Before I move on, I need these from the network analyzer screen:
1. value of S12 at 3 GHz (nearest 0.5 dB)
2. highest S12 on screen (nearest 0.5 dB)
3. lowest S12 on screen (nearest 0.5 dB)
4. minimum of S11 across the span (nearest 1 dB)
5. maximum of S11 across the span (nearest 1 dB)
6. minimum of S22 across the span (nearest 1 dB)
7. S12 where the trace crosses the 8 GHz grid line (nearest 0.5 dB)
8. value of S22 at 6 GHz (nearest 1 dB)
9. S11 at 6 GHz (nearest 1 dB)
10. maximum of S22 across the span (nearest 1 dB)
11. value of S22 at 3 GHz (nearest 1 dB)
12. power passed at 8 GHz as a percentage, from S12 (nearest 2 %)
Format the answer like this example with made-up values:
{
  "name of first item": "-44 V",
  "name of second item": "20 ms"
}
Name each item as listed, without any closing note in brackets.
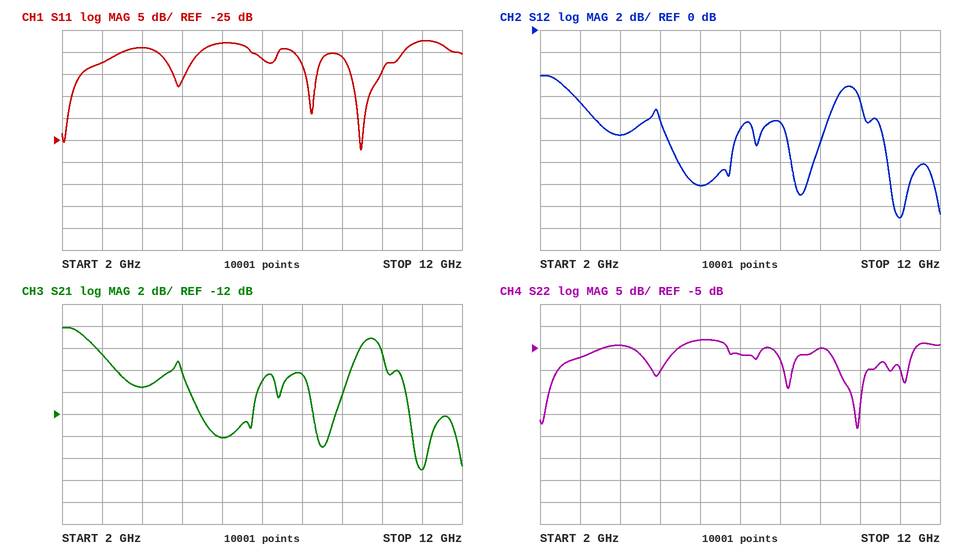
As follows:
{
  "value of S12 at 3 GHz": "-6.5 dB",
  "highest S12 on screen": "-4.0 dB",
  "lowest S12 on screen": "-17.0 dB",
  "minimum of S11 across the span": "-27 dB",
  "maximum of S11 across the span": "-2 dB",
  "minimum of S22 across the span": "-23 dB",
  "S12 where the trace crosses the 8 GHz grid line": "-8.5 dB",
  "value of S22 at 6 GHz": "-3 dB",
  "S11 at 6 GHz": "-3 dB",
  "maximum of S22 across the span": "-3 dB",
  "value of S22 at 3 GHz": "-7 dB",
  "power passed at 8 GHz as a percentage, from S12": "14 %"
}
